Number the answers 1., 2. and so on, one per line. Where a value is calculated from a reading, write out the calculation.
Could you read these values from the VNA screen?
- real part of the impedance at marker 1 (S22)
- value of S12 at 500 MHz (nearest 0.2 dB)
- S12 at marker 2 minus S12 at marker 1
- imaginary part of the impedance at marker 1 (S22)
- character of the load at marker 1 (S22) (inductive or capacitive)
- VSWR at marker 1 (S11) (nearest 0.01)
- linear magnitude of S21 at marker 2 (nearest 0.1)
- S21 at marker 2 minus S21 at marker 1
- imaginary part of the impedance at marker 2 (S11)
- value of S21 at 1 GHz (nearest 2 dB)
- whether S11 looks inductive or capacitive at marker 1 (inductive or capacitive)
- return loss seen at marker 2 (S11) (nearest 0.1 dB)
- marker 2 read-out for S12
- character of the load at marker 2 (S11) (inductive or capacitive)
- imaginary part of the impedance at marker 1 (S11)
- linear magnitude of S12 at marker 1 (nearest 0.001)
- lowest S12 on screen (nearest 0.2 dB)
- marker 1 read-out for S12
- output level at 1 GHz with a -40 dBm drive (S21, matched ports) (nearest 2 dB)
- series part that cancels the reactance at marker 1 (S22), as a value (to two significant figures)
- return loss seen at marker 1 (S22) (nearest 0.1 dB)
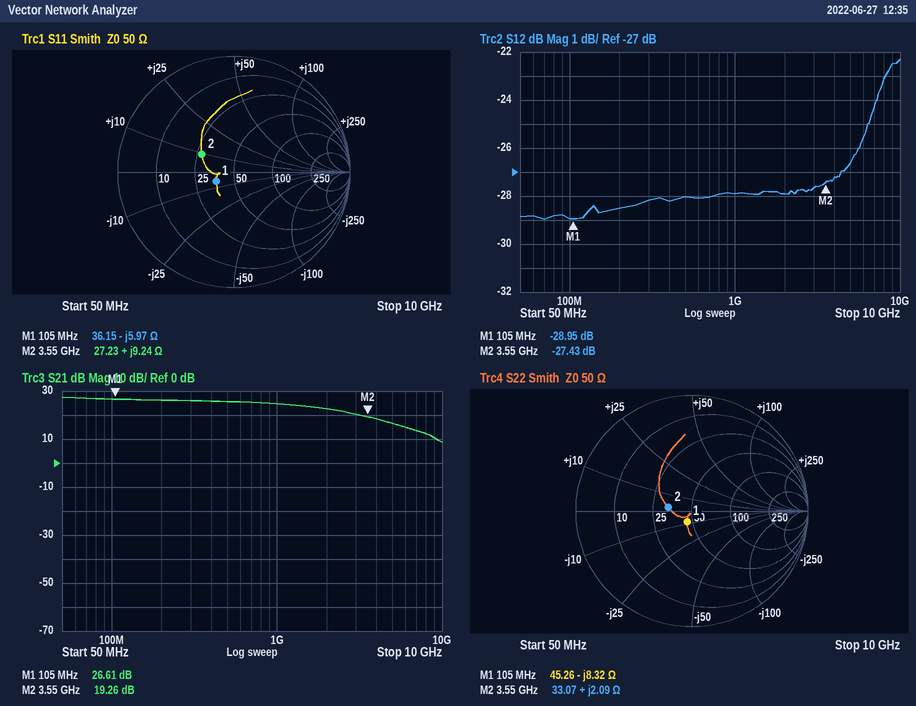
1. 45.26 Ω
2. -28.0 dB
3. -27.43 − (-28.95) = 1.52 dB
4. -8.32 Ω
5. capacitive
6. 1.42
7. 10^(19.26/20) ≈ 9.2
8. 19.26 − (26.61) = -7.35 dB
9. +9.24 Ω
10. 24 dB
11. capacitive
12. 10.0 dB
13. -27.43 dB
14. inductive
15. -5.97 Ω
16. 10^(-28.95/20) ≈ 0.036
17. -29.0 dB
18. -28.95 dB
19. -40 dBm + (24 dB) = -16 dBm
20. L = 8.32 Ω/(2π × 105 MHz) ≈ 13 nH
21. 20.0 dB
